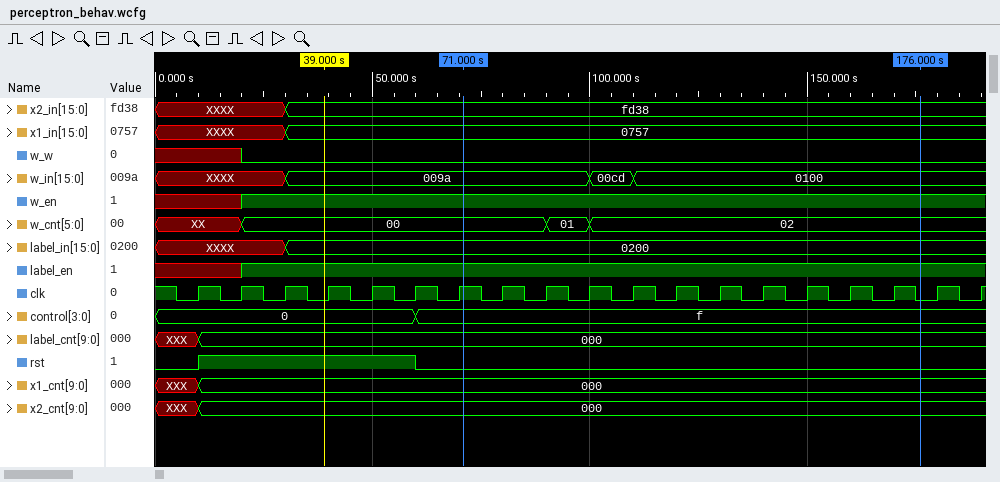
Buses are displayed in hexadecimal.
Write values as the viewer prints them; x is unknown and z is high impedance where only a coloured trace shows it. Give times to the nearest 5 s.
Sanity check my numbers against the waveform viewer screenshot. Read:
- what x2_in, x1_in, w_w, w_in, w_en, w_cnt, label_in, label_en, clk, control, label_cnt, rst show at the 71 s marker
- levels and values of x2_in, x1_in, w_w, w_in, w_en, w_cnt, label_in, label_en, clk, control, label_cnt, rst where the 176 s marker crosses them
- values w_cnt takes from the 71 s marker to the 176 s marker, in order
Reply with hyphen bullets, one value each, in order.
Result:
- x2_in=fd38, x1_in=0757, w_w=0, w_in=009a, w_en=1, w_cnt=00, label_in=0200, label_en=1, clk=1, control=f, label_cnt=000, rst=0
- x2_in=fd38, x1_in=0757, w_w=0, w_in=0100, w_en=1, w_cnt=02, label_in=0200, label_en=1, clk=0, control=f, label_cnt=000, rst=0
- 00, 01, 02
